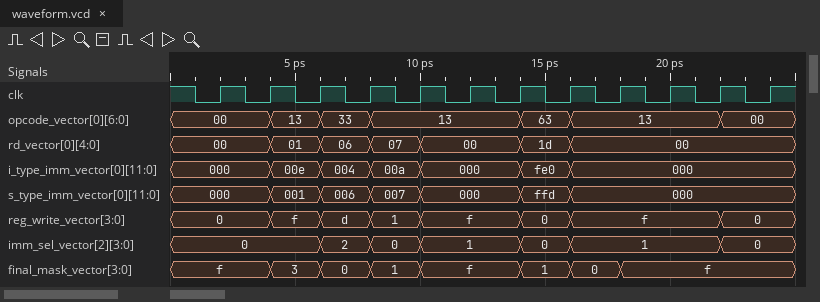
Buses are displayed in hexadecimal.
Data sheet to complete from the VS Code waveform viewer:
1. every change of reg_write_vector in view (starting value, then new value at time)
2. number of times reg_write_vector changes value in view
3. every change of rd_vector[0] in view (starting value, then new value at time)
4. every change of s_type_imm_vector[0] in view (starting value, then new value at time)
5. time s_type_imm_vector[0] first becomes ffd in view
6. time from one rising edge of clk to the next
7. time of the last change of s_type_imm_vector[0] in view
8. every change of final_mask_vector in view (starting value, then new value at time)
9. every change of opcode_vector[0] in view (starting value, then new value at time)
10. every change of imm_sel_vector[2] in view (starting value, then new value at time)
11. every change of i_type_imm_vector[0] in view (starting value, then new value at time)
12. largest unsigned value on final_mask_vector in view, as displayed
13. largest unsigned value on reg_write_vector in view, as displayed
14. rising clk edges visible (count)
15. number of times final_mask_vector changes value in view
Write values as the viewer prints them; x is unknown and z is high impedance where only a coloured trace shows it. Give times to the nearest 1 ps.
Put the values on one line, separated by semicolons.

0, f at 4 ps, d at 6 ps, 1 at 8 ps, f at 10 ps, 0 at 14 ps, f at 16 ps, 0 at 22 ps; 7; 00, 01 at 4 ps, 06 at 6 ps, 07 at 8 ps, 00 at 10 ps, 1d at 14 ps, 00 at 16 ps; 000, 001 at 4 ps, 006 at 6 ps, 007 at 8 ps, 000 at 10 ps, ffd at 14 ps, 000 at 16 ps; 14 ps; 2 ps; 16 ps; f, 3 at 4 ps, 0 at 6 ps, 1 at 8 ps, f at 10 ps, 1 at 14 ps, 0 at 16 ps, f at 18 ps; 00, 13 at 4 ps, 33 at 6 ps, 13 at 8 ps, 63 at 14 ps, 13 at 16 ps, 00 at 22 ps; 0, 2 at 6 ps, 0 at 8 ps, 1 at 10 ps, 0 at 14 ps, 1 at 16 ps, 0 at 22 ps; 000, 00e at 4 ps, 004 at 6 ps, 00a at 8 ps, 000 at 10 ps, fe0 at 14 ps, 000 at 16 ps; f; f; 12; 7
